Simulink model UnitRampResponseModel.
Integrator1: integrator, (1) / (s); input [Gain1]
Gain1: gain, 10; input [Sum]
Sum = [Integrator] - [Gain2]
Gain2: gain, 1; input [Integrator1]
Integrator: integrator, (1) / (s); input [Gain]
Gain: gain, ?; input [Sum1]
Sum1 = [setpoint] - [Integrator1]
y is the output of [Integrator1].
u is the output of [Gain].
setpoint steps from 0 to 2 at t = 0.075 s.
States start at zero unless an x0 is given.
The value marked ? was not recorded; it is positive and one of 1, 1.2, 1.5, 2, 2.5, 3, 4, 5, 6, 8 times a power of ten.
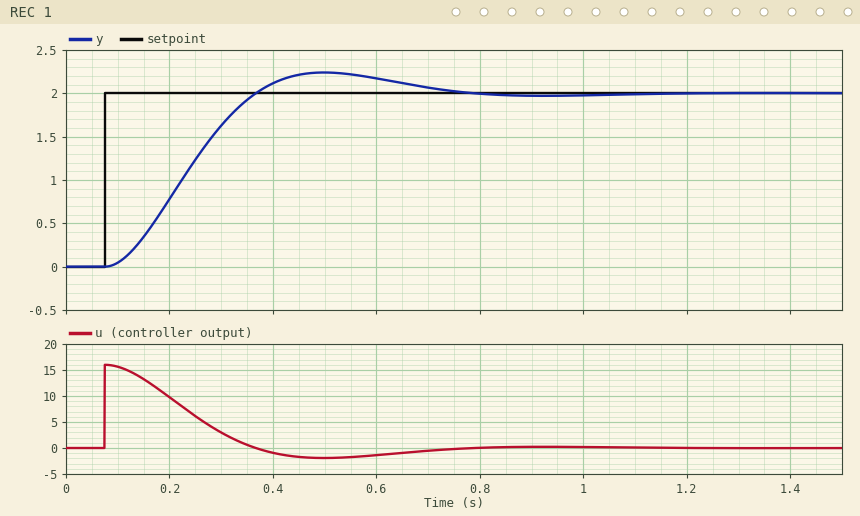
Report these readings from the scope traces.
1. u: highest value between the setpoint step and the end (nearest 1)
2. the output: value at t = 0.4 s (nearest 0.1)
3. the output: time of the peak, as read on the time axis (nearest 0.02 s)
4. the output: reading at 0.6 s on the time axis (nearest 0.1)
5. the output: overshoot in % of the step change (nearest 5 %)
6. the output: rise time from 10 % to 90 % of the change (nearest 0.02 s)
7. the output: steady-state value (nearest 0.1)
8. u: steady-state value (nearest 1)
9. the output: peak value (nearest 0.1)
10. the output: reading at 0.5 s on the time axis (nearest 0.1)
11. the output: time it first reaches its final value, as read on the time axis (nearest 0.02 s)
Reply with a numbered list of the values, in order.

1. 16
2. 2.1
3. 0.50 s
4. 2.2
5. 10 %
6. 0.20 s
7. 2.0
8. 0
9. 2.2
10. 2.2
11. 0.36 s
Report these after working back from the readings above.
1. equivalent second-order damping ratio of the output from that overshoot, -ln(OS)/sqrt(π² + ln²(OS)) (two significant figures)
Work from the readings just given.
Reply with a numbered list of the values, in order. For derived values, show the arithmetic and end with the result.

1. ln(0.1) = -2.303; 2.303 / sqrt(9.870 + 5.302) = 0.59
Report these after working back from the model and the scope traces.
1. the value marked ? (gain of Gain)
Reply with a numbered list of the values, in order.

1. 8
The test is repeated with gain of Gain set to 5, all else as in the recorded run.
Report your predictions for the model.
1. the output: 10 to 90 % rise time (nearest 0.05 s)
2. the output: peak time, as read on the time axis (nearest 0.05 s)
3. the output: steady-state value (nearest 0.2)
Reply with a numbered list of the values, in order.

1. 0.30 s
2. 0.70 s
3. 2.0
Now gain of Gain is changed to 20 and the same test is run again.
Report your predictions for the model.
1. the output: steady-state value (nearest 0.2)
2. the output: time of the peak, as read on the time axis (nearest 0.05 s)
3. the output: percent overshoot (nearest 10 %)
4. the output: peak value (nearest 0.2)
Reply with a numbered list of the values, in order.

1. 2.0
2. 0.30 s
3. 30 %
4. 2.6
